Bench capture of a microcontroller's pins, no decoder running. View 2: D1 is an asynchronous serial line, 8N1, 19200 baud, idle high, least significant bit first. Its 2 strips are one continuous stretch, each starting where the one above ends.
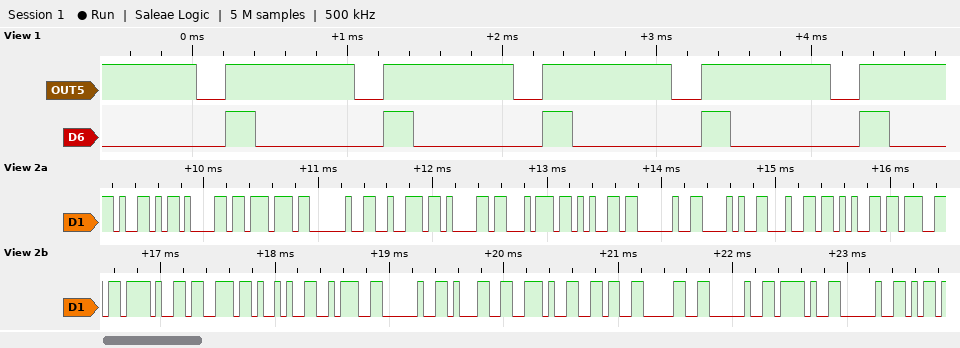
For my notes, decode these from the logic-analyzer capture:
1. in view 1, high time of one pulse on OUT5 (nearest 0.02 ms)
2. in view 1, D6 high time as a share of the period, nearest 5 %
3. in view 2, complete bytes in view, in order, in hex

0.84 ms
20 %
59 61 77 20 72 61 74 65 20 28 64 65 67 2F 73 29 3A 20 31 2E 36 30 20 2F 20
